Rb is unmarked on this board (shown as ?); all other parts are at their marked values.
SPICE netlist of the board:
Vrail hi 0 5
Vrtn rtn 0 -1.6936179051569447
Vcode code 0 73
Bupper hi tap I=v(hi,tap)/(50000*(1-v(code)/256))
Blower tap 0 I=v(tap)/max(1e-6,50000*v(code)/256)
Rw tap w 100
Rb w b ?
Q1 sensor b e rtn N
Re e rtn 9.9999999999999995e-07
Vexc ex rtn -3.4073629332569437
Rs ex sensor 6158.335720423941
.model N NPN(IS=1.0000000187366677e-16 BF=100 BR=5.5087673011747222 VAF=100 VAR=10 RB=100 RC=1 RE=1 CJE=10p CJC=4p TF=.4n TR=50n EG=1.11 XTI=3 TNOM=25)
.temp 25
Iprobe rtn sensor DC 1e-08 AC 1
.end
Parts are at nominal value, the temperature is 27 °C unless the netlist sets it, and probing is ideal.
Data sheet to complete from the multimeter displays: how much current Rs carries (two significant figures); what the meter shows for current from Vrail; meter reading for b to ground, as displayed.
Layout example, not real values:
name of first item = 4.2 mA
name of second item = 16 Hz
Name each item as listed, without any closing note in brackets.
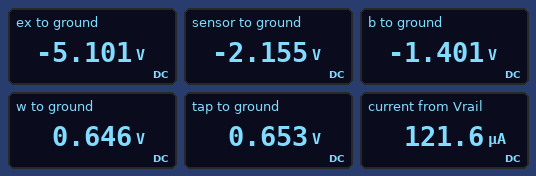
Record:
how much current Rs carries = 480 µA
what the meter shows for current from Vrail = 121.6 µA
meter reading for b to ground, as displayed = -1.401 V
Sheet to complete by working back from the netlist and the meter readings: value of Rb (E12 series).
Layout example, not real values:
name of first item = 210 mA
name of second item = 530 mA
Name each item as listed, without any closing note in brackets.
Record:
value of Rb = 27 kΩ
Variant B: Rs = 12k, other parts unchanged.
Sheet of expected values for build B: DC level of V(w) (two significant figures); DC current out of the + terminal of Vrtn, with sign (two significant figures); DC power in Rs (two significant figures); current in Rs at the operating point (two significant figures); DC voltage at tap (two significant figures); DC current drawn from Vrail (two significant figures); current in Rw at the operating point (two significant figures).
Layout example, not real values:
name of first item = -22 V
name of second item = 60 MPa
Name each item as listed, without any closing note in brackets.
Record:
DC level of V(w) = 760 mV
DC current out of the + terminal of Vrtn, with sign = -64 µA
DC power in Rs = 950 µW
current in Rs at the operating point = 280 µA
DC voltage at tap = 770 mV
DC current drawn from Vrail = 120 µA
current in Rw at the operating point = 64 µA
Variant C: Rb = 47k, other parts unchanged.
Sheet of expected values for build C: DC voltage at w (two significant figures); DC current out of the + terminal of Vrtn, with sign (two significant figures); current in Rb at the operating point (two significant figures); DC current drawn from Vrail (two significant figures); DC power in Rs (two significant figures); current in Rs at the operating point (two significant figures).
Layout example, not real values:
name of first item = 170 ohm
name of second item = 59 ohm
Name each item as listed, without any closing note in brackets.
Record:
DC voltage at w = 820 mV
DC current out of the + terminal of Vrtn, with sign = -59 µA
current in Rb at the operating point = 59 µA
DC current drawn from Vrail = 120 µA
DC power in Rs = 940 µW
current in Rs at the operating point = 390 µA
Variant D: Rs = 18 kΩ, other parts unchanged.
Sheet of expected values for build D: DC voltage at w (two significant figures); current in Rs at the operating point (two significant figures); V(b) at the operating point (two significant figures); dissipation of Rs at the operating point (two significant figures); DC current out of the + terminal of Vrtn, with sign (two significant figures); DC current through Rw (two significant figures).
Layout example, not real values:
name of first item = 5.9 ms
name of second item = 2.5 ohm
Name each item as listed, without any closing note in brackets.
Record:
DC voltage at w = 770 mV
current in Rs at the operating point = 190 µA
V(b) at the operating point = -960 mV
dissipation of Rs at the operating point = 640 µW
DC current out of the + terminal of Vrtn, with sign = -64 µA
DC current through Rw = 64 µA
